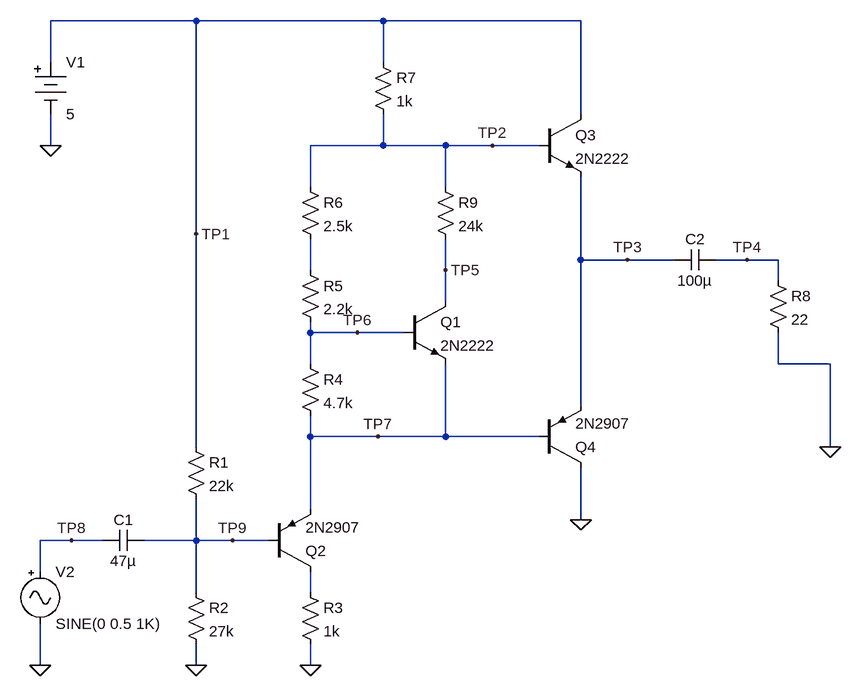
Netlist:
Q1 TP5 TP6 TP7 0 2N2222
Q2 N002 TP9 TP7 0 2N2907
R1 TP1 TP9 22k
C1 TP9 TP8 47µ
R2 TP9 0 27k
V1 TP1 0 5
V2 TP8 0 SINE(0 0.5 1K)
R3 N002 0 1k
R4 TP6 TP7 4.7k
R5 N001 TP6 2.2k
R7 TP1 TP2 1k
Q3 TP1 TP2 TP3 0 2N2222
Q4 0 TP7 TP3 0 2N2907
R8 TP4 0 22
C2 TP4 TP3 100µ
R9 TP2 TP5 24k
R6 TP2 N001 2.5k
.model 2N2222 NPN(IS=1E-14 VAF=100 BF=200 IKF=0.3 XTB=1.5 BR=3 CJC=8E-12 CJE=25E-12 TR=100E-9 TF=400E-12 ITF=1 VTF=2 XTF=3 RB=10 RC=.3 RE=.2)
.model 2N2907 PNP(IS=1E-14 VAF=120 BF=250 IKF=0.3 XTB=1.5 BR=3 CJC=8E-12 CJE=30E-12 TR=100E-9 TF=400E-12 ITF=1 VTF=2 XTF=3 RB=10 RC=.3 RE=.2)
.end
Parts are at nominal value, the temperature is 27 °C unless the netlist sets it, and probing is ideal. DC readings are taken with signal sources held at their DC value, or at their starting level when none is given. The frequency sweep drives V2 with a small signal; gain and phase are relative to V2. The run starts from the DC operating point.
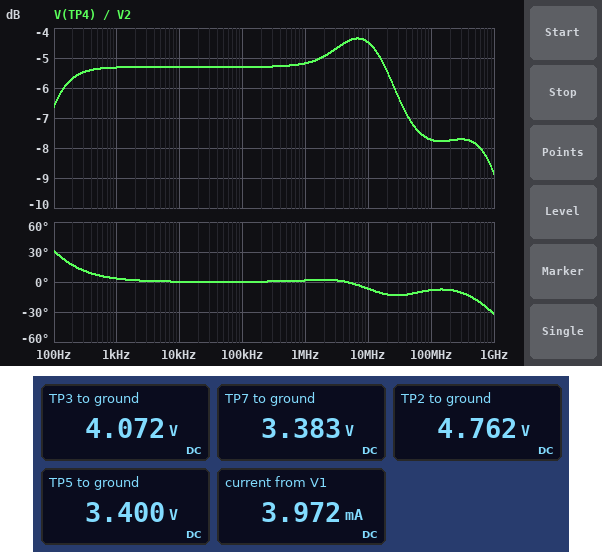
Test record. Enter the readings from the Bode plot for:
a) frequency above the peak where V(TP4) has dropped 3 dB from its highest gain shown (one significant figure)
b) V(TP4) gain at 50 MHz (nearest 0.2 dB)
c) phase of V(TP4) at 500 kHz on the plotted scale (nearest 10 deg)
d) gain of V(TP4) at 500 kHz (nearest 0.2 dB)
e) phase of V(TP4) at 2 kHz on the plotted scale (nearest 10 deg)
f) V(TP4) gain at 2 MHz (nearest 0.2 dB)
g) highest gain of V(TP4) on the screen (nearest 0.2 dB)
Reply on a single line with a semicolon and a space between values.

60 MHz; -7.2 dB; 0 deg; -5.2 dB; 0 deg; -5.0 dB; -4.4 dB
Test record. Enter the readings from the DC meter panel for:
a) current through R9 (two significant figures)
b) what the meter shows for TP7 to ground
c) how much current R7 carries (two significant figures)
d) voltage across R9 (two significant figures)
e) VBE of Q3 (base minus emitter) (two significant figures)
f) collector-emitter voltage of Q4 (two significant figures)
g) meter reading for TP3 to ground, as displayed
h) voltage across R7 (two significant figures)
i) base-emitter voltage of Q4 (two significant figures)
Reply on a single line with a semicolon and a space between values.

57 µA; 3.383 V; 240 µA; 1.4 V; 690 mV; -4.1 V; 4.072 V; 240 mV; -690 mV
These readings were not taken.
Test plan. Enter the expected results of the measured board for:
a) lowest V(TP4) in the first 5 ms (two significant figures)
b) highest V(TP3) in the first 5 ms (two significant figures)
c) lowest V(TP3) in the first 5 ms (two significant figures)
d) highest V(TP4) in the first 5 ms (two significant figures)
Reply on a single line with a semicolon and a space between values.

-370 mV; 4.2 V; 3.7 V; 150 mV
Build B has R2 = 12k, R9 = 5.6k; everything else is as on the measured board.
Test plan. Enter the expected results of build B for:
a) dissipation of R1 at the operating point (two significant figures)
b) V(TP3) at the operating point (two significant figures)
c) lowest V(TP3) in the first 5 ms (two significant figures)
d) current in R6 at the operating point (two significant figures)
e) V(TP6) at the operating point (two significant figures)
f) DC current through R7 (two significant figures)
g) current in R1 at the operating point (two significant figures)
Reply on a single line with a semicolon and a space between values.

470 µW; 3.2 V; 2.8 V; 200 µA; 3.1 V; 970 µA; 150 µA
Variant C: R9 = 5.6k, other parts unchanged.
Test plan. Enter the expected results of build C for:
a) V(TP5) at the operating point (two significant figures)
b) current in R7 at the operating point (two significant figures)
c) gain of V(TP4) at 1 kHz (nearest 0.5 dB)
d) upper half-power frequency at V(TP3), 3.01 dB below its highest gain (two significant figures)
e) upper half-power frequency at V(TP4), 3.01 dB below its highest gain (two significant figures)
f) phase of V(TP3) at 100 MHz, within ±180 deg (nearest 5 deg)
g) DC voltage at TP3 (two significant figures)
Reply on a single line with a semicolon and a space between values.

3.5 V; 350 µA; -12.5 dB; 31 Hz; 1.8 GHz; 25 deg; 4.0 V
